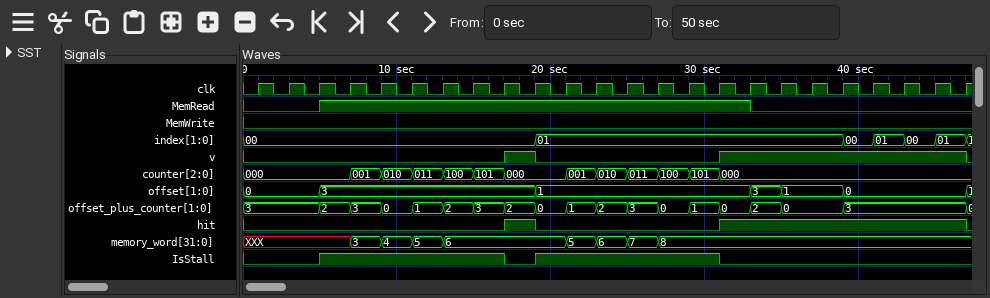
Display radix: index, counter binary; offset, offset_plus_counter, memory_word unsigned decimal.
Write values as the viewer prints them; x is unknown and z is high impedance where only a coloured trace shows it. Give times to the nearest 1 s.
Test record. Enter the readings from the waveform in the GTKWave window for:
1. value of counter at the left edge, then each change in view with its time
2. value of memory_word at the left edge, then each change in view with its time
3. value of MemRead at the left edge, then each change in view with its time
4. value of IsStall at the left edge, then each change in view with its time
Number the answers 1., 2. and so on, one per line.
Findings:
1. 000, 001 at 7 s, 010 at 9 s, 011 at 11 s, 100 at 13 s, 101 at 15 s, 000 at 17 s, 001 at 21 s, 010 at 23 s, 011 at 25 s, 100 at 27 s, 101 at 29 s, 000 at 31 s
2. XXX, 3 at 7 s, 4 at 9 s, 5 at 11 s, 6 at 13 s, 5 at 21 s, 6 at 23 s, 7 at 25 s, 8 at 27 s
3. 0, 1 at 5 s, 0 at 33 s
4. 0, 1 at 5 s, 0 at 17 s, 1 at 19 s, 0 at 31 s
